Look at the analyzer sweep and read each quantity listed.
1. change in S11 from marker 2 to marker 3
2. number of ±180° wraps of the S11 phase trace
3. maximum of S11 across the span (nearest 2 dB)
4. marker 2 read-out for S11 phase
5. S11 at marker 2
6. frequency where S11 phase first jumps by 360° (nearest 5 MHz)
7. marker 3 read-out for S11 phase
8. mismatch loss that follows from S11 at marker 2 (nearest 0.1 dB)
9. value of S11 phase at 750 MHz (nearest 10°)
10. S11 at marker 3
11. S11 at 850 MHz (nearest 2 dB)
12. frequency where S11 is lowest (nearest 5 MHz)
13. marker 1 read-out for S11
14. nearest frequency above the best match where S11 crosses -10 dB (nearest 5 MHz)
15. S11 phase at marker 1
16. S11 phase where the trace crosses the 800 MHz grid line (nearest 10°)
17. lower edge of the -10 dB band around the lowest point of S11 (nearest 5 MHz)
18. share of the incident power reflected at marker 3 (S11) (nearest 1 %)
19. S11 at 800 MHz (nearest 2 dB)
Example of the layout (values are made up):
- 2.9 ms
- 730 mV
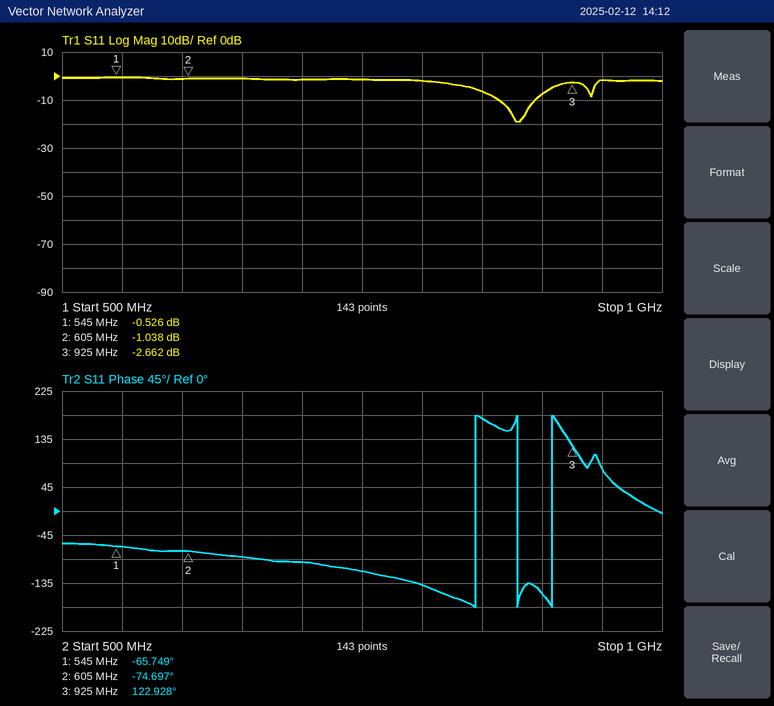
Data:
- -1.624 dB
- 3
- 0 dB
- -74.697°
- -1.038 dB
- 845 MHz
- 122.928°
- 6.7 dB
- -110°
- -2.662 dB
- -6 dB
- 880 MHz
- -0.526 dB
- 895 MHz
- -65.749°
- -140°
- 865 MHz
- 54 %
- -2 dB
